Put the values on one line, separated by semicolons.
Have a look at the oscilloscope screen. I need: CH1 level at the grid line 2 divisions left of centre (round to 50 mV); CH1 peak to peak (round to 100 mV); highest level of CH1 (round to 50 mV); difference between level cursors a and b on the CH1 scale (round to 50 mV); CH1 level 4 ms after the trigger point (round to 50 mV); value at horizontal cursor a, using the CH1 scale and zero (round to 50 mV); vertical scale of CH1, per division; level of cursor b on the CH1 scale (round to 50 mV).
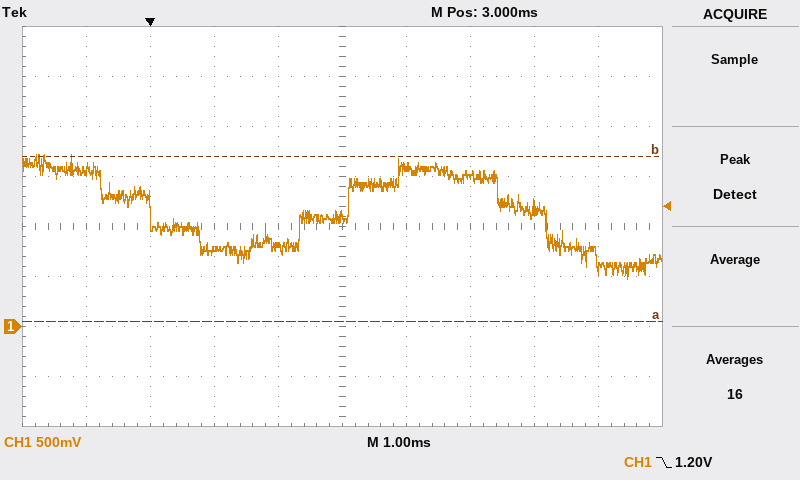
750 mV; 1.20 V; 1.70 V; 1.65 V; 1.60 V; 50 mV; 500 mV; 1.70 V
